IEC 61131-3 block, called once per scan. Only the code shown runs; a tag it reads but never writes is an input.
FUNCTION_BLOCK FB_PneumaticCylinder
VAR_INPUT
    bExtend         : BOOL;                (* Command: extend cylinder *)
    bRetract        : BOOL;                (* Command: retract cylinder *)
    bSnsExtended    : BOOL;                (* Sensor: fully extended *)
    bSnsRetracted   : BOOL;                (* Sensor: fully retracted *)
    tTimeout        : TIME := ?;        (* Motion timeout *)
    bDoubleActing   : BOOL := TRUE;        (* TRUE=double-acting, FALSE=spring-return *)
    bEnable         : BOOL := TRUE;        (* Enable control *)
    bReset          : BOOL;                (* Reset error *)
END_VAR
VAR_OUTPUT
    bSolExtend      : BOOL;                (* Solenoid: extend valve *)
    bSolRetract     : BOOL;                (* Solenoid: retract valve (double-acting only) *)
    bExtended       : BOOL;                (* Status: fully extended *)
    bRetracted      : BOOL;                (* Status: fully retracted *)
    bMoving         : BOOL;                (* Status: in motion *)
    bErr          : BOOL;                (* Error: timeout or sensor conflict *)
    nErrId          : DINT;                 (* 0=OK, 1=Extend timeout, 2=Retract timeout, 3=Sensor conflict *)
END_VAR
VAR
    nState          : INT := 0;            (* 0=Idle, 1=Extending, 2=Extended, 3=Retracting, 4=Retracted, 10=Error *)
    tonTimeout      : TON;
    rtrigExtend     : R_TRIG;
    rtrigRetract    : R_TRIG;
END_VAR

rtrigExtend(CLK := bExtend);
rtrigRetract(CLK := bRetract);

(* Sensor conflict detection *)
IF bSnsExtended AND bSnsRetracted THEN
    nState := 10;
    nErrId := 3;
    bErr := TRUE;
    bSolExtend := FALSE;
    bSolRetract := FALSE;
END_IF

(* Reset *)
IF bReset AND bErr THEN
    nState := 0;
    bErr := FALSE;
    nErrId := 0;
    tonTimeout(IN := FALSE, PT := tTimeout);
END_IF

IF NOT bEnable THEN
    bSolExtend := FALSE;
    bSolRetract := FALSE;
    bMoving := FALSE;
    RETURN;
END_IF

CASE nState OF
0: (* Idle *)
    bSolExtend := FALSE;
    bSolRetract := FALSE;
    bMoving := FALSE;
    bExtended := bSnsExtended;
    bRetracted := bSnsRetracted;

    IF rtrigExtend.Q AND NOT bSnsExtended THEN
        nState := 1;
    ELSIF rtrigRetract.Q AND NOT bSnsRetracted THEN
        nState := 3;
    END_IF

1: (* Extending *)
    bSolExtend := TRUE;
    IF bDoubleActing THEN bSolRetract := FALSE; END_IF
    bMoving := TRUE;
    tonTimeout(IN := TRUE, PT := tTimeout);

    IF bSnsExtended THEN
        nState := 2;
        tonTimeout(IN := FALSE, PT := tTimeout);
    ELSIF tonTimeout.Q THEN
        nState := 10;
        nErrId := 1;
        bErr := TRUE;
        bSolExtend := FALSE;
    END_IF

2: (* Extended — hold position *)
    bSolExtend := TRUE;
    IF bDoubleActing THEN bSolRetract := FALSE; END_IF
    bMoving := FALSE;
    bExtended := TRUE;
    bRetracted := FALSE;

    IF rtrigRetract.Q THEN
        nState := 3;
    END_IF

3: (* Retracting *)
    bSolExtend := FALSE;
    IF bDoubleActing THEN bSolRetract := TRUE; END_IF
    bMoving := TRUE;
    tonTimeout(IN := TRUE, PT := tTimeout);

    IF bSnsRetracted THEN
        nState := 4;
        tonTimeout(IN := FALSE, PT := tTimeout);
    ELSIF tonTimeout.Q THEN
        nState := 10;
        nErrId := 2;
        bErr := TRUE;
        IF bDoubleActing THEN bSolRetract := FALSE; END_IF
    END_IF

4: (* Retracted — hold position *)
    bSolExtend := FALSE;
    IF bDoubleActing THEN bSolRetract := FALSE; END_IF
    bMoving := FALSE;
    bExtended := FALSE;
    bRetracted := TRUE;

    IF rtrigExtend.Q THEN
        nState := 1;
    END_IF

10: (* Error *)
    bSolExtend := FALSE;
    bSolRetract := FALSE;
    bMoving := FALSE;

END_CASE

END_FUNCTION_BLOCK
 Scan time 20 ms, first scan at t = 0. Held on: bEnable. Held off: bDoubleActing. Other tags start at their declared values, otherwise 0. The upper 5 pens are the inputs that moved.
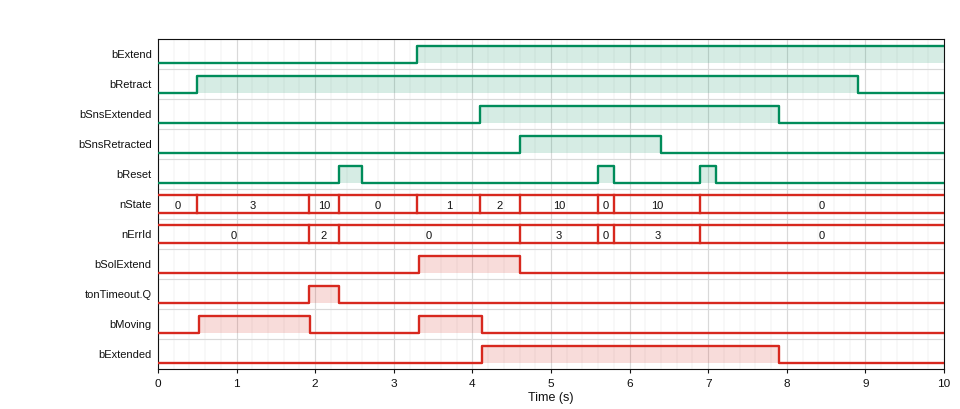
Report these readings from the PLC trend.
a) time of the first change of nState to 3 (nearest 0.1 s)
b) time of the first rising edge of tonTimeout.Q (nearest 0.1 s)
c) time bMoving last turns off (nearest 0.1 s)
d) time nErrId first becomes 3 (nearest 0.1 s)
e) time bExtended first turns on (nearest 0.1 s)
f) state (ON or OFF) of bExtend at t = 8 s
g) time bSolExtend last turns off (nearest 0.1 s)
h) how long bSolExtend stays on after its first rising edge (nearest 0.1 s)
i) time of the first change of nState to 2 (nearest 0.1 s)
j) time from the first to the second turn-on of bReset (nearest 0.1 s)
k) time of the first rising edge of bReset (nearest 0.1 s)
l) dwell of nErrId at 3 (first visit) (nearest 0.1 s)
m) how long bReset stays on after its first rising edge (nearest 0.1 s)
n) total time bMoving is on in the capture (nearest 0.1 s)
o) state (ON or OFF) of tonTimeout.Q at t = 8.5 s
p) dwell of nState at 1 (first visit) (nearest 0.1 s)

0.5 s
1.9 s
4.1 s
4.6 s
4.1 s
ON
4.6 s
1.3 s
4.1 s
3.3 s
2.3 s
1.0 s
0.3 s
2.2 s
OFF
0.8 s
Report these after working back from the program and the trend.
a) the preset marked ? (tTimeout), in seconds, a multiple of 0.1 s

1.4 s
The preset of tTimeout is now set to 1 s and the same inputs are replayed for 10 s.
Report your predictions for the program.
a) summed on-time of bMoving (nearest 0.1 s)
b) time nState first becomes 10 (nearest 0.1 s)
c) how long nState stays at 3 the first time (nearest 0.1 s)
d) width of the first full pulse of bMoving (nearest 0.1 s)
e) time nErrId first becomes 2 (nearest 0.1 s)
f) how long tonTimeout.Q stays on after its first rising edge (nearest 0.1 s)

1.8 s
1.5 s
1.0 s
1.0 s
1.5 s
0.8 s
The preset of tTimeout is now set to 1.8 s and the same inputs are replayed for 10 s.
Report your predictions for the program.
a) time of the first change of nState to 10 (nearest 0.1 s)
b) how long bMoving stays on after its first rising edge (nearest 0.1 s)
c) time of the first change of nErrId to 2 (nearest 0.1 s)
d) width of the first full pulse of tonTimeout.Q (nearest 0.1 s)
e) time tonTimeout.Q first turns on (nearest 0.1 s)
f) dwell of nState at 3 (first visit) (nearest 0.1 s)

2.3 s
1.8 s
2.3 s
0.0 s
2.3 s
1.8 s
